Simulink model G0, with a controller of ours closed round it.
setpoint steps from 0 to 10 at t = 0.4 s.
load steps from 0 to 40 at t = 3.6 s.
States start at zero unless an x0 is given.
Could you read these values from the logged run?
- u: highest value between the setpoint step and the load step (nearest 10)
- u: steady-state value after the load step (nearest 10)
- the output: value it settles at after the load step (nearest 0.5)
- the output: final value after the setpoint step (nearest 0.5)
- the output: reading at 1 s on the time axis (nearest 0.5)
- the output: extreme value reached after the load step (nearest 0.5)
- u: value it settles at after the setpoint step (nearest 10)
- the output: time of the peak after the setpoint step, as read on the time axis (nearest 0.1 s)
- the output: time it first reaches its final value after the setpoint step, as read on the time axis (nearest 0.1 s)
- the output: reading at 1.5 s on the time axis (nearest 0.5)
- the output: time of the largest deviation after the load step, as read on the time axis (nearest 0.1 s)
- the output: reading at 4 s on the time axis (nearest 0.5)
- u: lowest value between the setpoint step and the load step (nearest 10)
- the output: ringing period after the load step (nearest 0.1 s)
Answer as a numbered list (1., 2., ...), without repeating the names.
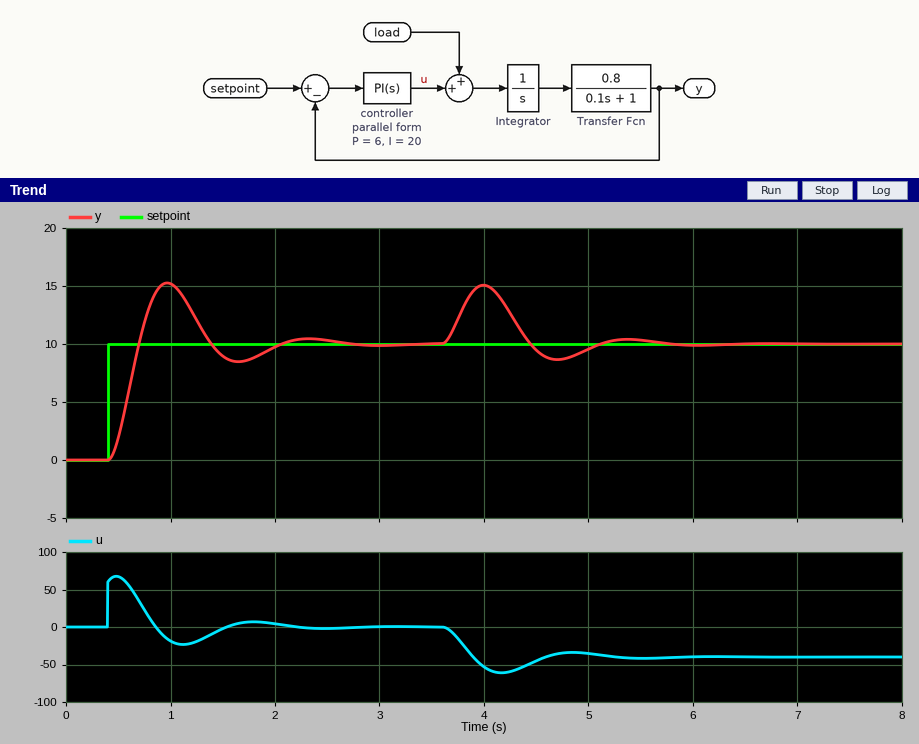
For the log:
1. 70
2. -40
3. 10.0
4. 10.0
5. 15.0
6. 15.0
7. 0
8. 1.0 s
9. 0.7 s
10. 9.0
11. 4.0 s
12. 15.0
13. -20
14. 1.4 s
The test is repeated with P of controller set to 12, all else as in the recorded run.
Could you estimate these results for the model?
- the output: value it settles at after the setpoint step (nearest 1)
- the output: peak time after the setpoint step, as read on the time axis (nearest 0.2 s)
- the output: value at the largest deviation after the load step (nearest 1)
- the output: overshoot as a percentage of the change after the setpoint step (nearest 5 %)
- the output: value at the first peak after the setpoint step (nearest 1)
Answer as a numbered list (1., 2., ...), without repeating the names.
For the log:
1. 10
2. 0.8 s
3. 13
4. 35 %
5. 14
